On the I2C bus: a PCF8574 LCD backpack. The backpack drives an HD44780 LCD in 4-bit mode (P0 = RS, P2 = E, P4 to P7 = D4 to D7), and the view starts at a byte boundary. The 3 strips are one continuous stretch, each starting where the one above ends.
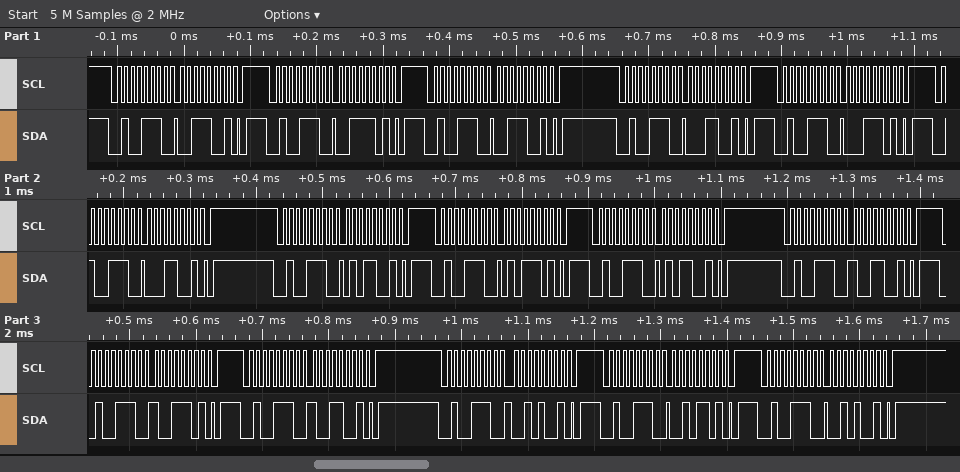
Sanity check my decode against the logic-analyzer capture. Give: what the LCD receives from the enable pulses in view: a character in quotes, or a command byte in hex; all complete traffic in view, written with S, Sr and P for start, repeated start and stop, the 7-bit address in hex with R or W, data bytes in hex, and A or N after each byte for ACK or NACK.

'1' 'Y'
S 27W A 39 A P S 27W A 3D A P S 27W A 39 A P S 27W A 19 A P S 27W A 1D A P S 27W A 19 A P S 27W A 59 A P S 27W A 5D A P S 27W A 59 A P S 27W A 99 A P S 27W A 9D A P S 27W A 99 A P S 27W A 29 A P S 27W A 2D A P S 27W A 29 A P
